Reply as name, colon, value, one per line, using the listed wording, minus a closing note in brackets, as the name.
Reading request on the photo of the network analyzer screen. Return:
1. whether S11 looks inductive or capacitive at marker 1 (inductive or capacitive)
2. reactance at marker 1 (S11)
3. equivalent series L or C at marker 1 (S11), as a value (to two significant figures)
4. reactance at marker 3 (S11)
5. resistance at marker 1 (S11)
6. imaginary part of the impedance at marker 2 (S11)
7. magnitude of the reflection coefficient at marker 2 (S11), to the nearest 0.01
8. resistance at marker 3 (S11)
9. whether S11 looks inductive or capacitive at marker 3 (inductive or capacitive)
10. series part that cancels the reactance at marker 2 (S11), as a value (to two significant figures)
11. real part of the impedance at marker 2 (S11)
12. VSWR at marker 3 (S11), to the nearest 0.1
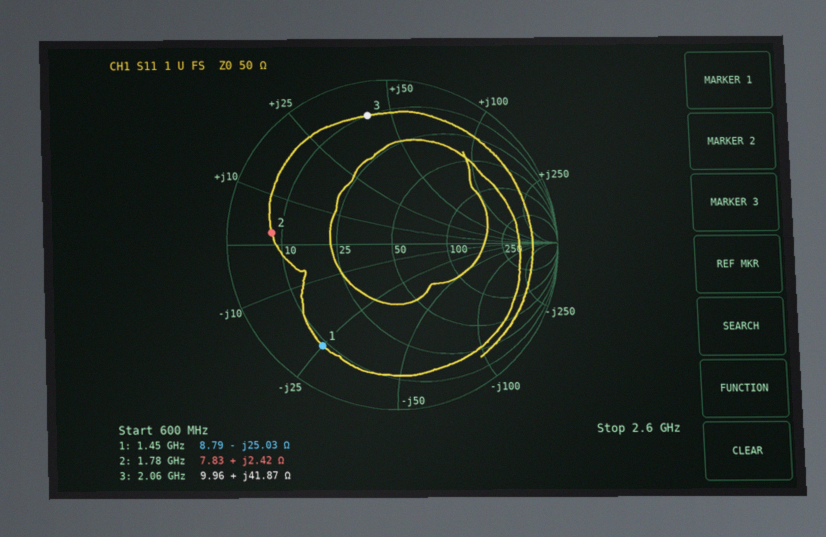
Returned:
whether S11 looks inductive or capacitive at marker 1: capacitive
reactance at marker 1: -25.03 Ω
equivalent series L or C at marker 1 (S11), as a value: 4.4 pF
reactance at marker 3: +41.87 Ω
resistance at marker 1: 8.79 Ω
imaginary part of the impedance at marker 2: +2.42 Ω
magnitude of the reflection coefficient at marker 2 (S11), to the nearest 0.01: 0.73
resistance at marker 3: 9.96 Ω
whether S11 looks inductive or capacitive at marker 3: inductive
series part that cancels the reactance at marker 2 (S11), as a value: 37 pF
real part of the impedance at marker 2: 7.83 Ω
VSWR at marker 3 (S11), to the nearest 0.1: 8.6
